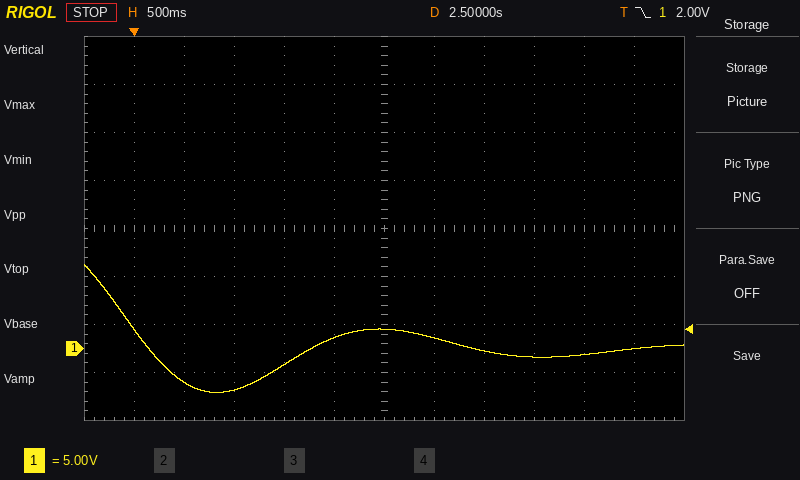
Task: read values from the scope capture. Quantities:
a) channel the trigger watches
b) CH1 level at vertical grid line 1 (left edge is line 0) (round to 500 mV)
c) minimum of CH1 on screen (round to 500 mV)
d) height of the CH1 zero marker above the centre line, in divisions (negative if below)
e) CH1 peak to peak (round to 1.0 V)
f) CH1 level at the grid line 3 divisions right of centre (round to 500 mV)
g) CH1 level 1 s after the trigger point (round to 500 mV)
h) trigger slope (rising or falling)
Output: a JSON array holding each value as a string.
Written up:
["CH1", "2.0 V", "-4.5 V", "-2.5 div", "13.0 V", "-1.0 V", "-4.5 V", "falling"]
